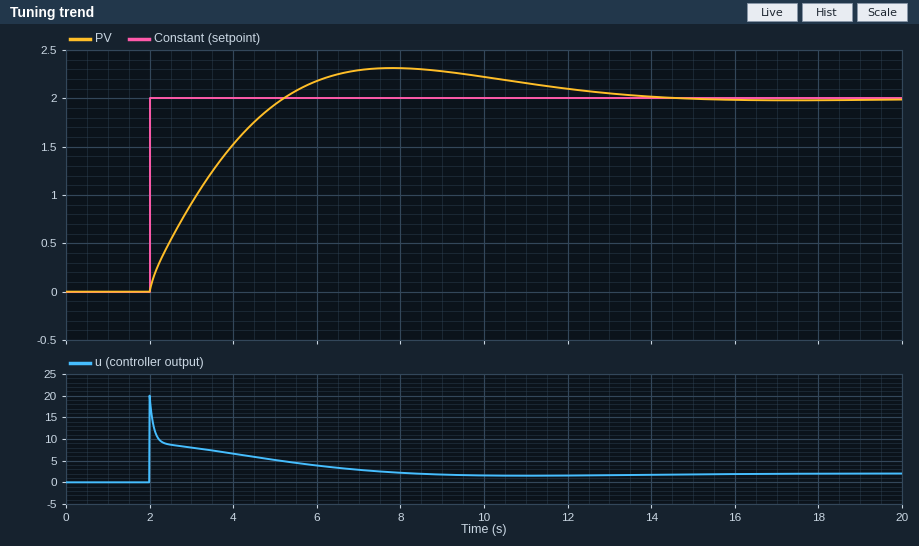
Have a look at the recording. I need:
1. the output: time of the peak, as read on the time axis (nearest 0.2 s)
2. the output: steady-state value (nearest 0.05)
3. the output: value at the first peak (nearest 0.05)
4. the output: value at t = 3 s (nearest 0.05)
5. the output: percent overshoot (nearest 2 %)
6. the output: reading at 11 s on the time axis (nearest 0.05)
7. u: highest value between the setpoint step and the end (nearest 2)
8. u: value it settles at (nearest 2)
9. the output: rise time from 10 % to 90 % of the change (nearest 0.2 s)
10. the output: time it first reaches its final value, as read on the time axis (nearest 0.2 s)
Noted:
7.8 s
2.00
2.30
0.90
16 %
2.15
20
2
2.4 s
5.2 s
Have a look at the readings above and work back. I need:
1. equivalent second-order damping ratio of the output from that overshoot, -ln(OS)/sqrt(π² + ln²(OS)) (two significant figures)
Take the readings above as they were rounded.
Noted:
0.50
